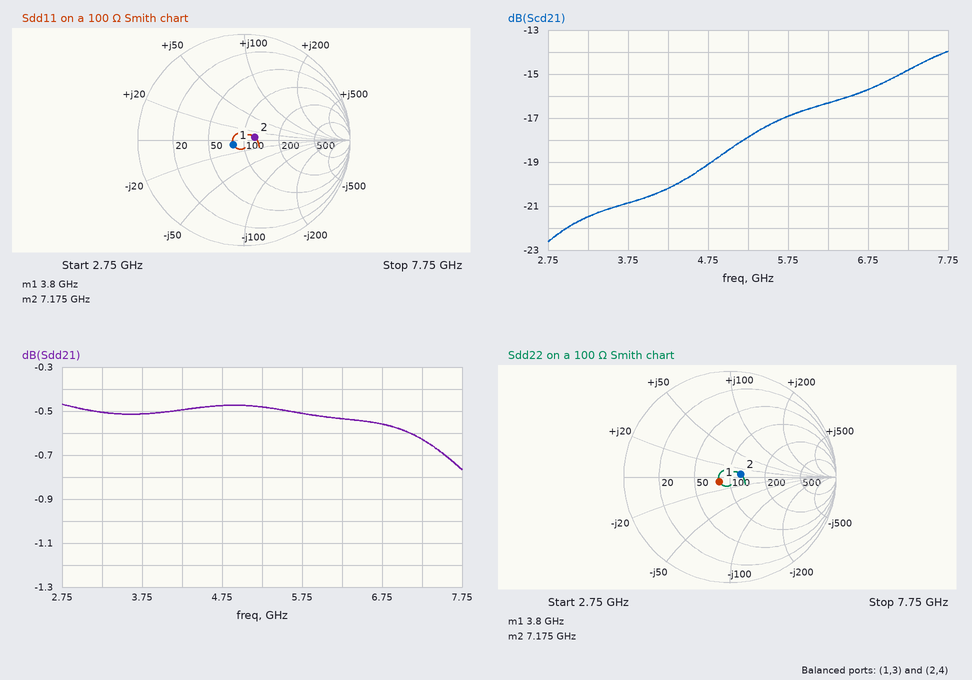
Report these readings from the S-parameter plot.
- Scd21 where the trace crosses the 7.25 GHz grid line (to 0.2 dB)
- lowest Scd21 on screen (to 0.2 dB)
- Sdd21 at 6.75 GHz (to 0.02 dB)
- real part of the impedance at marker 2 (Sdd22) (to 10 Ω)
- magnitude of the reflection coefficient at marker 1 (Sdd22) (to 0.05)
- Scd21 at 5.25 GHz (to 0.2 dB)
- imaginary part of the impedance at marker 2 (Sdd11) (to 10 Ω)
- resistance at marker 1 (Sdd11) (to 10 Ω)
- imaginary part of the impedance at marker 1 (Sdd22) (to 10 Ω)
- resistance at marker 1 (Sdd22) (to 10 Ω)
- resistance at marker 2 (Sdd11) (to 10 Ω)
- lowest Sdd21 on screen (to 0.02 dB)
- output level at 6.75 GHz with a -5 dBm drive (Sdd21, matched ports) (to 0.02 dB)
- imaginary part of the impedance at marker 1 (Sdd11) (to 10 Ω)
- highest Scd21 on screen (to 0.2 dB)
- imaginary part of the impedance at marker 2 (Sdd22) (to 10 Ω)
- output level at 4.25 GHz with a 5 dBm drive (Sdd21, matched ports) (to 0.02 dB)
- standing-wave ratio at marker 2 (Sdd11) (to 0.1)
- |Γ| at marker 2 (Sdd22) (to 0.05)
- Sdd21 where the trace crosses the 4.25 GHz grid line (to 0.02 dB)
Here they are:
-14.8 dB
-22.6 dB
-0.56 dB
120 Ω
0.10
-17.8 dB
+10 Ω
80 Ω
-10 Ω
80 Ω
120 Ω
-0.76 dB
-5.56 dBm
-10 Ω
-14.0 dB
+10 Ω
4.50 dBm
1.2
0.10
-0.50 dB
